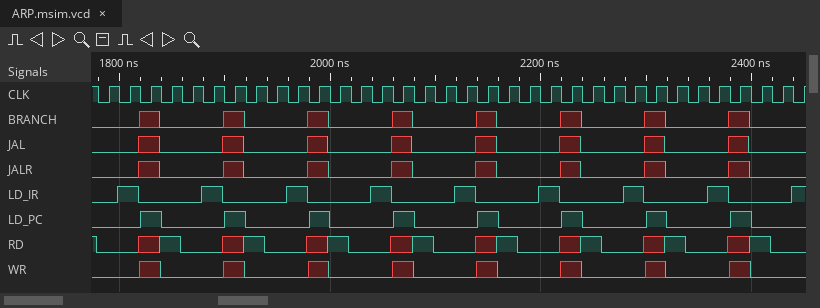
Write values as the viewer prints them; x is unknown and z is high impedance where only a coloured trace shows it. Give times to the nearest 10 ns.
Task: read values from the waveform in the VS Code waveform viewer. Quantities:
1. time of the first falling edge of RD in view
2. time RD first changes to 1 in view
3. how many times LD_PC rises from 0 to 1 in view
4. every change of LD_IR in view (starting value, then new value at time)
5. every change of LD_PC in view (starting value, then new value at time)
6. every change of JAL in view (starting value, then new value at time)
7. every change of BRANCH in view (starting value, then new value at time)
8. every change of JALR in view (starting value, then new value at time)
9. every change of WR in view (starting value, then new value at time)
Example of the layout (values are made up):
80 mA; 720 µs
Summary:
1780 ns; 1840 ns; 8; 0, 1 at 1800 ns, 0 at 1820 ns, 1 at 1880 ns, 0 at 1900 ns, 1 at 1960 ns, 0 at 1980 ns, 1 at 2040 ns, 0 at 2060 ns, 1 at 2120 ns, 0 at 2140 ns, 1 at 2200 ns, 0 at 2220 ns, 1 at 2280 ns, 0 at 2300 ns, 1 at 2360 ns, 0 at 2380 ns, 1 at 2440 ns; 0, 1 at 1820 ns, 0 at 1840 ns, 1 at 1900 ns, 0 at 1920 ns, 1 at 1980 ns, 0 at 2000 ns, 1 at 2060 ns, 0 at 2080 ns, 1 at 2140 ns, 0 at 2160 ns, 1 at 2220 ns, 0 at 2240 ns, 1 at 2300 ns, 0 at 2320 ns, 1 at 2380 ns, 0 at 2400 ns; 0, x at 1820 ns, 0 at 1840 ns, x at 1900 ns, 0 at 1920 ns, x at 1980 ns, 0 at 2000 ns, x at 2060 ns, 0 at 2080 ns, x at 2140 ns, 0 at 2160 ns, x at 2220 ns, 0 at 2240 ns, x at 2300 ns, 0 at 2320 ns, x at 2380 ns, 0 at 2400 ns; 0, x at 1820 ns, 0 at 1840 ns, x at 1900 ns, 0 at 1920 ns, x at 1980 ns, 0 at 2000 ns, x at 2060 ns, 0 at 2080 ns, x at 2140 ns, 0 at 2160 ns, x at 2220 ns, 0 at 2240 ns, x at 2300 ns, 0 at 2320 ns, x at 2380 ns, 0 at 2400 ns; 0, x at 1820 ns, 0 at 1840 ns, x at 1900 ns, 0 at 1920 ns, x at 1980 ns, 0 at 2000 ns, x at 2060 ns, 0 at 2080 ns, x at 2140 ns, 0 at 2160 ns, x at 2220 ns, 0 at 2240 ns, x at 2300 ns, 0 at 2320 ns, x at 2380 ns, 0 at 2400 ns; 0, x at 1820 ns, 0 at 1840 ns, x at 1900 ns, 0 at 1920 ns, x at 1980 ns, 0 at 2000 ns, x at 2060 ns, 0 at 2080 ns, x at 2140 ns, 0 at 2160 ns, x at 2220 ns, 0 at 2240 ns, x at 2300 ns, 0 at 2320 ns, x at 2380 ns, 0 at 2400 ns
